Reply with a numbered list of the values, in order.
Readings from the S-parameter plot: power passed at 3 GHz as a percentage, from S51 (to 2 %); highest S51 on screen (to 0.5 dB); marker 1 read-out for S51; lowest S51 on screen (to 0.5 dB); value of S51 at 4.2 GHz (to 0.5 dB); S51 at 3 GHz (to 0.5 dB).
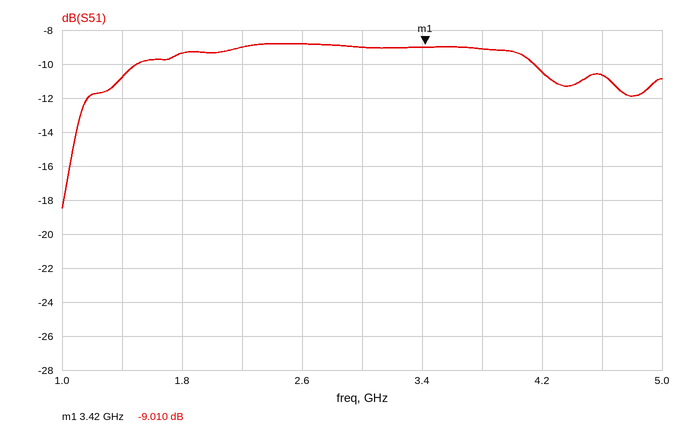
1. 12 %
2. -9.0 dB
3. -9.010 dB
4. -18.5 dB
5. -10.5 dB
6. -9.0 dB
